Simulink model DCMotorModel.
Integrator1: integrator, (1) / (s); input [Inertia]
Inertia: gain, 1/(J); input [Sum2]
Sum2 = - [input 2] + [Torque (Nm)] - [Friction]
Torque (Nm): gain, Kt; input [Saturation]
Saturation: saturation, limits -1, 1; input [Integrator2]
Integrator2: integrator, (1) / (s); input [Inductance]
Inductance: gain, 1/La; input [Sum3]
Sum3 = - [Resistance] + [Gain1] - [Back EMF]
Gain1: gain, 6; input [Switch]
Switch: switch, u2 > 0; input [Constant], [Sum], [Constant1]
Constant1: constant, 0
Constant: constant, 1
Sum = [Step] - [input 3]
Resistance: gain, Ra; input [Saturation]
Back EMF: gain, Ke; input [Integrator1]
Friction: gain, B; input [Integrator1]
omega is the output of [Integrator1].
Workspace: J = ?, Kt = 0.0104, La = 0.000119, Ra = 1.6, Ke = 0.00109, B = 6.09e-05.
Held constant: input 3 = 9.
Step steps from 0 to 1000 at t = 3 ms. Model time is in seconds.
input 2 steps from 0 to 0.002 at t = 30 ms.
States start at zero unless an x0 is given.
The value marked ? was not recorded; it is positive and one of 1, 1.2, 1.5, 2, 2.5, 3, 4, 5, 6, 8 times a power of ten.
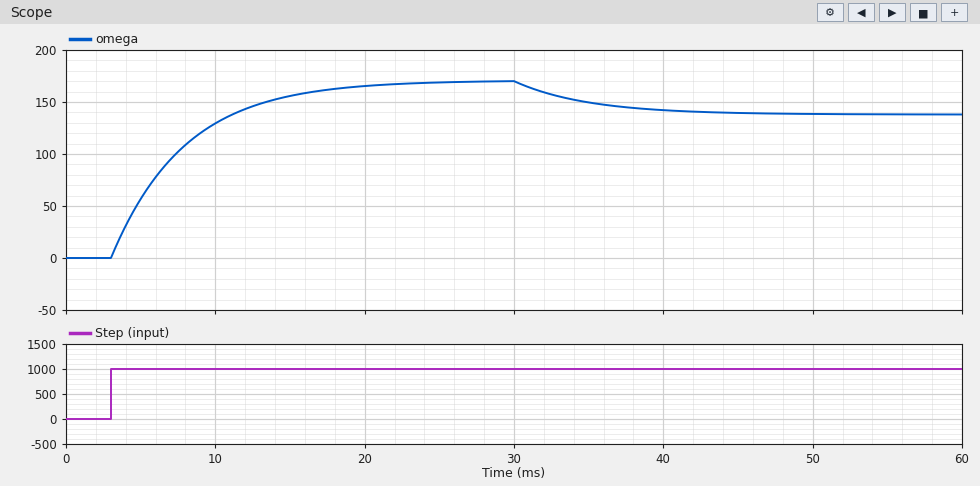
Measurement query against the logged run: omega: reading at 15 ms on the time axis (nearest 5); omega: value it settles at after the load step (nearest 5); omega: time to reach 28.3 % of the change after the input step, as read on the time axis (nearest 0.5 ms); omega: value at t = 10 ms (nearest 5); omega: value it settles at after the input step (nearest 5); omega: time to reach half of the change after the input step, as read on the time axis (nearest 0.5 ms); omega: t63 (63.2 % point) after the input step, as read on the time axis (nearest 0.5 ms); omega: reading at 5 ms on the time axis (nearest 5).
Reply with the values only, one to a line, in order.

155
140
4.5 ms
130
170
6.5 ms
8.0 ms
55
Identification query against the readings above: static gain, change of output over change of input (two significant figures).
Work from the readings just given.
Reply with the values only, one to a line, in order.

0.17
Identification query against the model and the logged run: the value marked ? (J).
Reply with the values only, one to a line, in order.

3e-07
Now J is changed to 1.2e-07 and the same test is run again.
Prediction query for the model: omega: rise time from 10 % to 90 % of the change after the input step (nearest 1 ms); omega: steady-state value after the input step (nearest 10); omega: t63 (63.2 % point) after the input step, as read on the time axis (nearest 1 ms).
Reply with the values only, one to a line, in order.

4 ms
170
5 ms
